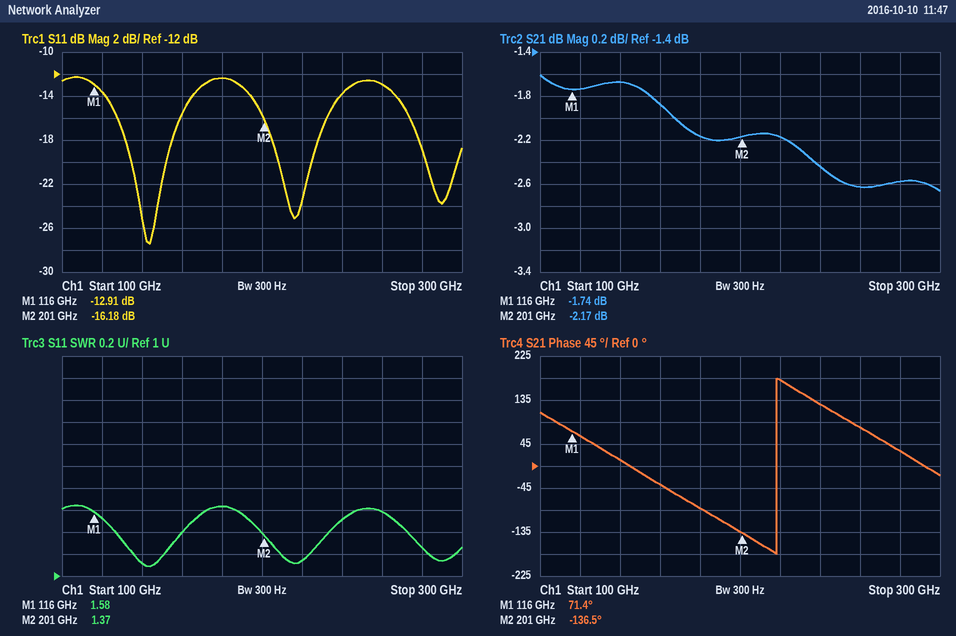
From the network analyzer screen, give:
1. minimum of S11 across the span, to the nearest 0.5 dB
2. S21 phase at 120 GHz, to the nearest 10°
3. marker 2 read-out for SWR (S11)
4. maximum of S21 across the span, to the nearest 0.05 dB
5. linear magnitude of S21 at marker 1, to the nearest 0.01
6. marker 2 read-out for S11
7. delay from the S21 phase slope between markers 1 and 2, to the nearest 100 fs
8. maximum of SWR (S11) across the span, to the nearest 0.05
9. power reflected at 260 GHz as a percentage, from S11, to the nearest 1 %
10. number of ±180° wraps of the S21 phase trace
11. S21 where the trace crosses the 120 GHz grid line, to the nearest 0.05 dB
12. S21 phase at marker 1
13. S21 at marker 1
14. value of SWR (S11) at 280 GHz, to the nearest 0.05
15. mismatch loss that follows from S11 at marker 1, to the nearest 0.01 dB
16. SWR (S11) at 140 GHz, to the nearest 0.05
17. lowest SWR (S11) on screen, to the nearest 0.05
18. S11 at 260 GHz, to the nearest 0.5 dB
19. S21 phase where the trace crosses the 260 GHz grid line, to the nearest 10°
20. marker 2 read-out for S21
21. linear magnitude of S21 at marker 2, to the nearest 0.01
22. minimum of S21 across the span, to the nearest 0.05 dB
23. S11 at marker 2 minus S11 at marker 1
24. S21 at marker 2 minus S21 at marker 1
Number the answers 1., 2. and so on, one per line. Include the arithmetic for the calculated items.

1. -27.5 dB
2. 60°
3. 1.37
4. -1.60 dB
5. 10^(-1.74/20) ≈ 0.82
6. -16.18 dB
7. −(-136.5° − (71.4°))/(360° × 85 GHz) ≈ 6.8 ps
8. 1.65
9. 10^(-13/10) ≈ 5 %
10. 1
11. -1.75 dB
12. 71.4°
13. -1.74 dB
14. 1.25
15. −10 log10(1 − 10^(-12.91/10)) ≈ 0.23 dB
16. 1.10
17. 1.10
18. -13.0 dB
19. 80°
20. -2.17 dB
21. 10^(-2.17/20) ≈ 0.78
22. -2.65 dB
23. -16.18 − (-12.91) = -3.27 dB
24. -2.17 − (-1.74) = -0.43 dB
